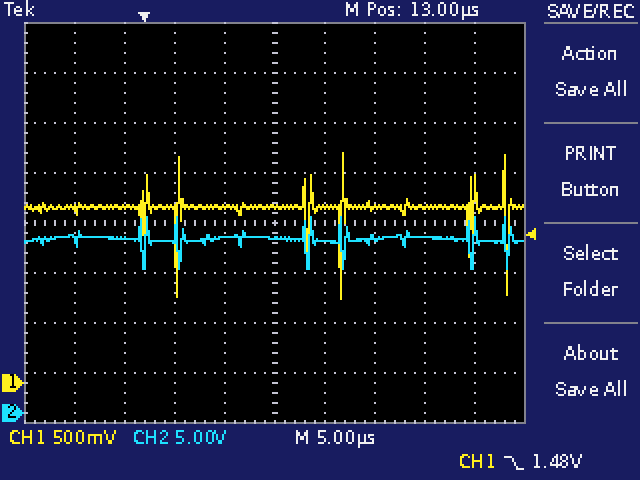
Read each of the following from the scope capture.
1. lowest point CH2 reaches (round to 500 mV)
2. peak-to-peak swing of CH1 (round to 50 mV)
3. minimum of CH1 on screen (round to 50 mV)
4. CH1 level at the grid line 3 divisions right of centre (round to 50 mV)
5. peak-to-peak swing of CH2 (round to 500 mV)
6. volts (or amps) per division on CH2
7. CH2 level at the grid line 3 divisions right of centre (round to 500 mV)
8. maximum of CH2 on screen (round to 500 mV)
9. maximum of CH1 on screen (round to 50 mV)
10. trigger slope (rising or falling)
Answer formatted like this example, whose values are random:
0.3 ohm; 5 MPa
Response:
14.5 V; 1.45 V; 850 mV; 1.75 V; 5.0 V; 5 V; 17.5 V; 19.5 V; 2.30 V; falling
